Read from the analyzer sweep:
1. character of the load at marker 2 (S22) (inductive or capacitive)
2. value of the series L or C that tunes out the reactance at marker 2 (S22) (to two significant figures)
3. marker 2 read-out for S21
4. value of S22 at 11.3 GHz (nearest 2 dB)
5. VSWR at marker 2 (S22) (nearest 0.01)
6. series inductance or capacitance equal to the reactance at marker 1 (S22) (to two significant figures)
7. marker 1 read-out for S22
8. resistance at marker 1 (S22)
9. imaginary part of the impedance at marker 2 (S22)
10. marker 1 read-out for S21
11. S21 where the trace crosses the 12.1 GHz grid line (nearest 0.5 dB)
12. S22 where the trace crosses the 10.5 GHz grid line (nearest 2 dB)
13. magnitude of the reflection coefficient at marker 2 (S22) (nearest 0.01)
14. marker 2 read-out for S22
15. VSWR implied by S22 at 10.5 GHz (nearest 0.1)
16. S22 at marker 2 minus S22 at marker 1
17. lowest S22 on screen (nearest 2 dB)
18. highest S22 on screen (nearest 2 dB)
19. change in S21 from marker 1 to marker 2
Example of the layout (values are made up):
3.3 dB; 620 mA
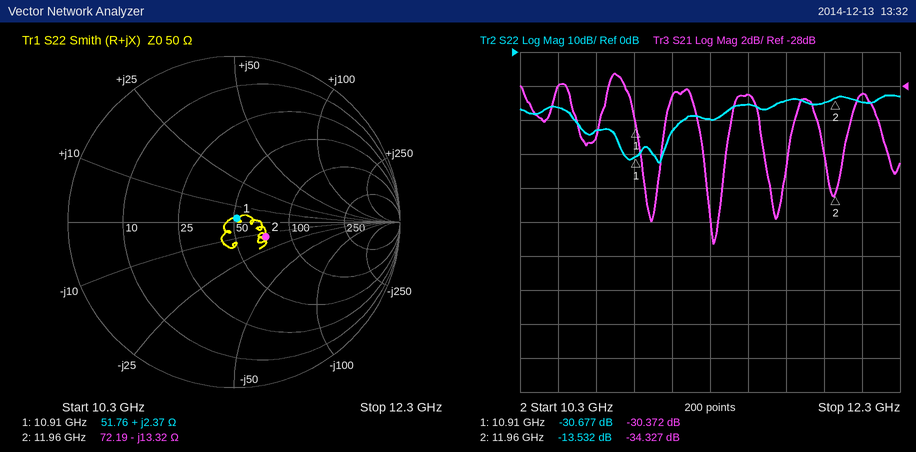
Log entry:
capacitive; 180 pH; -34.327 dB; -20 dB; 1.53; 35 pH; -30.677 dB; 51.76 Ω; -13.32 Ω; -30.372 dB; -28.5 dB; -16 dB; 0.21; -13.532 dB; 1.4; 17.145 dB; -32 dB; -12 dB; -3.955 dB
